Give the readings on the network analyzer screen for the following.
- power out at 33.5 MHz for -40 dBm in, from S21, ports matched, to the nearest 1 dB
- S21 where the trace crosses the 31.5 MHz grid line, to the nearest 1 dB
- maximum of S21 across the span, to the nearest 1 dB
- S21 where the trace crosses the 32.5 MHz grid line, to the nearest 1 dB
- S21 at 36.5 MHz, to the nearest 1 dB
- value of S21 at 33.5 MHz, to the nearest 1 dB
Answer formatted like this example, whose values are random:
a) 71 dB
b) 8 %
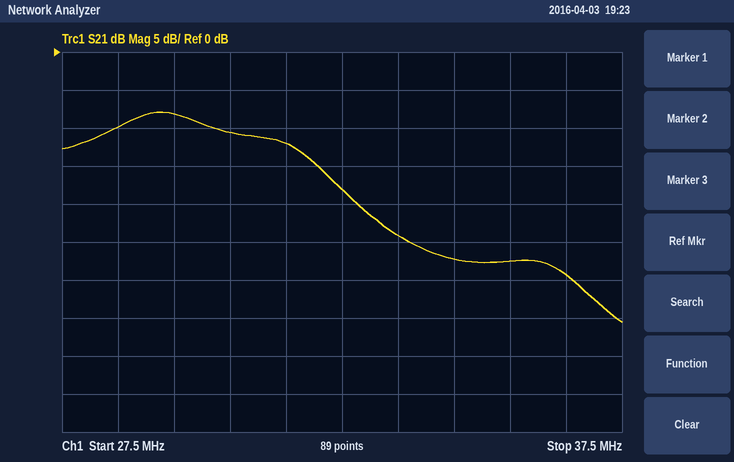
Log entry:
a) -64 dBm
b) -12 dB
c) -8 dB
d) -18 dB
e) -29 dB
f) -24 dB
